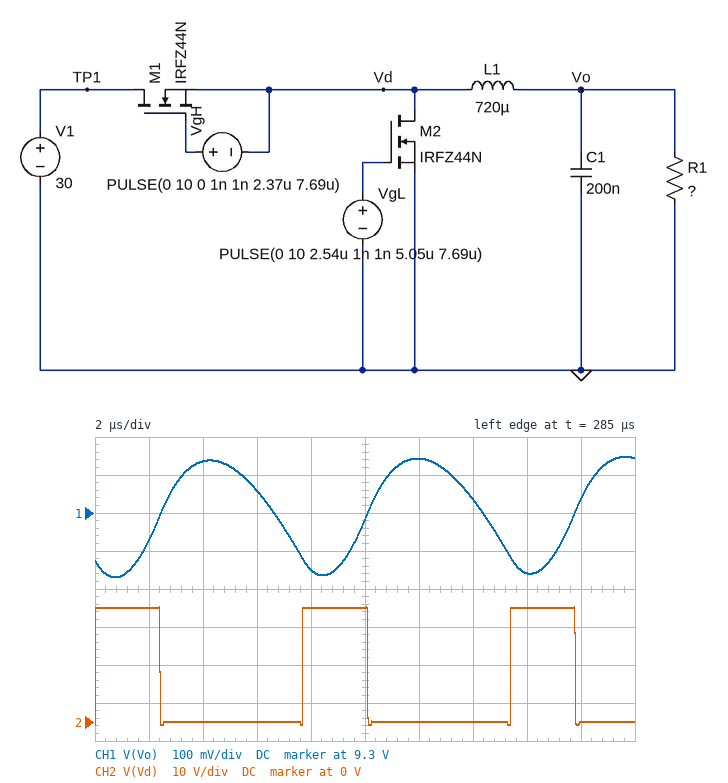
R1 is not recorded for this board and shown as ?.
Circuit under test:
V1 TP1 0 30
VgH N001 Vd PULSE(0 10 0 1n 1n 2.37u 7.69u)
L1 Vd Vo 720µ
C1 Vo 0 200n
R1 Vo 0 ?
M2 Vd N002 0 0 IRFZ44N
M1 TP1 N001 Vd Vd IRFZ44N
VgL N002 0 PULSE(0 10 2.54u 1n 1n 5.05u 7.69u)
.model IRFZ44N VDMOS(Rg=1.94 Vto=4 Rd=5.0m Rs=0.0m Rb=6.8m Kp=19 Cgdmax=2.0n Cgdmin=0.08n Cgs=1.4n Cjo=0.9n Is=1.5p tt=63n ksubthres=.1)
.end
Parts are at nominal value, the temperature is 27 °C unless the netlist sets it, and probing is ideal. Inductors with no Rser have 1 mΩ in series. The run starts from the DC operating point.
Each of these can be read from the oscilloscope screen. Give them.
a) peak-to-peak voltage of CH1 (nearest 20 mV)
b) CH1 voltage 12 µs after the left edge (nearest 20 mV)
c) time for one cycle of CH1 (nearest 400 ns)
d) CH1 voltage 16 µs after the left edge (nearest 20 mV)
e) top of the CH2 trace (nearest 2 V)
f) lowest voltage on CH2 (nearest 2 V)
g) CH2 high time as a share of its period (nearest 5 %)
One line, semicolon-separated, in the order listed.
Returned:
320 mV; 9.44 V; 7.6 µs; 9.14 V; 30 V; 0 V; 30 %
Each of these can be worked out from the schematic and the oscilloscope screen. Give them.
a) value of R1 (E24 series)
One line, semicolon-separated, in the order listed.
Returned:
13 Ω
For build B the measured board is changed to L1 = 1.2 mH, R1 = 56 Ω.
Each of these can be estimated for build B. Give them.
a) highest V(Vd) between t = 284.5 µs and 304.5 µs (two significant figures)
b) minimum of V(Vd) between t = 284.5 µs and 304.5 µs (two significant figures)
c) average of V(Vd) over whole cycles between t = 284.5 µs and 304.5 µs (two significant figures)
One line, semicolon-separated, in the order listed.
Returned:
31 V; -660 mV; 9.7 V
